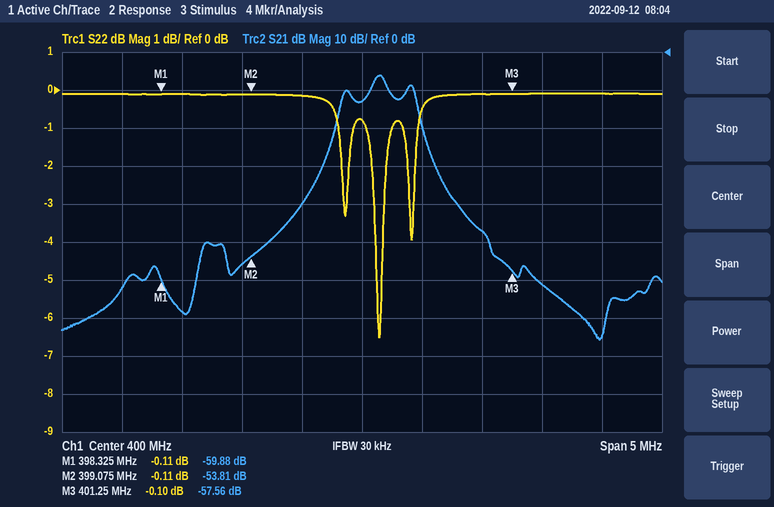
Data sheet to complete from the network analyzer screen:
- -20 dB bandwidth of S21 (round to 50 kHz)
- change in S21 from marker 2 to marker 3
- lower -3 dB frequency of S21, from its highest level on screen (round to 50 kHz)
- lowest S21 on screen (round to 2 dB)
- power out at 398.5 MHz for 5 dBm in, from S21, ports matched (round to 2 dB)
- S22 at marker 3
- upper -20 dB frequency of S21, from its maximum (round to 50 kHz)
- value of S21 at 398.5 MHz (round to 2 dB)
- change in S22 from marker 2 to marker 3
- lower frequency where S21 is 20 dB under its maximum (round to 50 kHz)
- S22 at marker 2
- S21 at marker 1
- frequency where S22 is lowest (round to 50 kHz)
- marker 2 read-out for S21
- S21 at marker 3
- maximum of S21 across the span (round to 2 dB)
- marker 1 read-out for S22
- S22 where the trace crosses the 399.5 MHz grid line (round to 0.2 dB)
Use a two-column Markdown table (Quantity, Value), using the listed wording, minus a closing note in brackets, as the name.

| Quantity | Value |
|---|---|
| -20 dB bandwidth of S21 | 850 kHz |
| change in S21 from marker 2 to marker 3 | -3.75 dB |
| lower -3 dB frequency of S21, from its highest level on screen | 400.10 MHz |
| lowest S21 on screen | -76 dB |
| power out at 398.5 MHz for 5 dBm in, from S21, ports matched | -64 dBm |
| S22 at marker 3 | -0.10 dB |
| upper -20 dB frequency of S21, from its maximum | 400.55 MHz |
| value of S21 at 398.5 MHz | -68 dB |
| change in S22 from marker 2 to marker 3 | 0.01 dB |
| lower frequency where S21 is 20 dB under its maximum | 399.70 MHz |
| S22 at marker 2 | -0.11 dB |
| S21 at marker 1 | -59.88 dB |
| frequency where S22 is lowest | 400.15 MHz |
| marker 2 read-out for S21 | -53.81 dB |
| S21 at marker 3 | -57.56 dB |
| maximum of S21 across the span | -6 dB |
| marker 1 read-out for S22 | -0.11 dB |
| S22 where the trace crosses the 399.5 MHz grid line | -0.2 dB |
